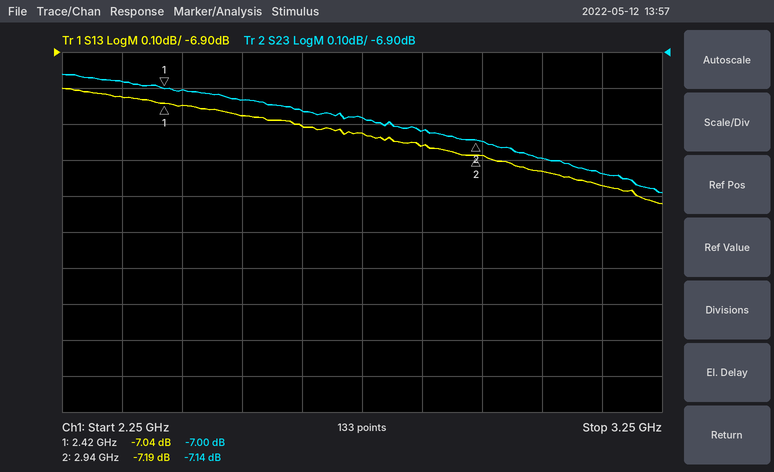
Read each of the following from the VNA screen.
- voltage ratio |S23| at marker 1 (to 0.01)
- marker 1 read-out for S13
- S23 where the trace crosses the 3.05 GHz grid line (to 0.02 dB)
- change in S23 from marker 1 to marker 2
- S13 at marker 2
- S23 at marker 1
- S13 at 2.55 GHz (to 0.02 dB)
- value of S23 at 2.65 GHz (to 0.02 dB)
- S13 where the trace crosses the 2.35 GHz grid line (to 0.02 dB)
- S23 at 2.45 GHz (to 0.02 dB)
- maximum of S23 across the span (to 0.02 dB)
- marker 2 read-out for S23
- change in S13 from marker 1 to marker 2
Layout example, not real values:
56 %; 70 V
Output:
0.45; -7.04 dB; -7.20 dB; -0.14 dB; -7.19 dB; -7.00 dB; -7.08 dB; -7.06 dB; -7.02 dB; -7.00 dB; -6.96 dB; -7.14 dB; -0.15 dB
